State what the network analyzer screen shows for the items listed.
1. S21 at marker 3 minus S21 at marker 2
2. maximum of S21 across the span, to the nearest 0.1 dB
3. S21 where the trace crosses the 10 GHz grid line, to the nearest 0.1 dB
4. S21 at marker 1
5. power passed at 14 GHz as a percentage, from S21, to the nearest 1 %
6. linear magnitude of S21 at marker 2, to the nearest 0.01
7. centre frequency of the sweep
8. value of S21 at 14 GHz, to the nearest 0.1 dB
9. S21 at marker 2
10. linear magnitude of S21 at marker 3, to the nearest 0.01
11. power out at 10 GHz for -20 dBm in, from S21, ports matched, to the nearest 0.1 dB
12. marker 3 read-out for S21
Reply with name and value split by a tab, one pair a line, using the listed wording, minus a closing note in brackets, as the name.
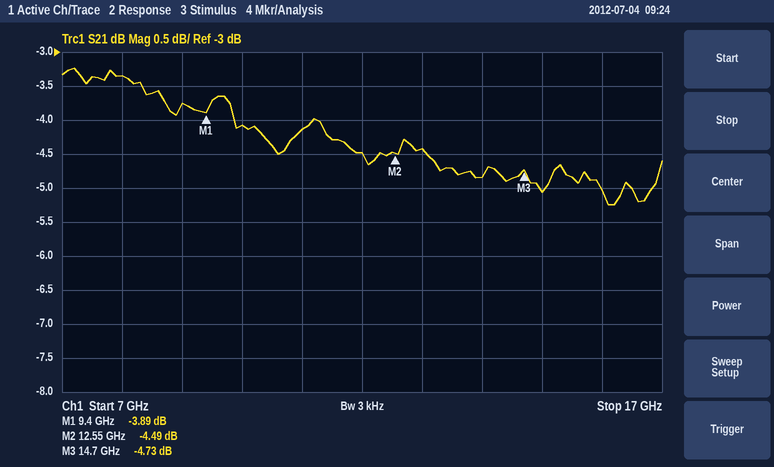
S21 at marker 3 minus S21 at marker 2	-0.24 dB
maximum of S21 across the span, to the nearest 0.1 dB	-3.2 dB
S21 where the trace crosses the 10 GHz grid line, to the nearest 0.1 dB	-4.1 dB
S21 at marker 1	-3.89 dB
power passed at 14 GHz as a percentage, from S21, to the nearest 1 %	33 %
linear magnitude of S21 at marker 2, to the nearest 0.01	0.60
centre frequency of the sweep	12 GHz
value of S21 at 14 GHz, to the nearest 0.1 dB	-4.8 dB
S21 at marker 2	-4.49 dB
linear magnitude of S21 at marker 3, to the nearest 0.01	0.58
power out at 10 GHz for -20 dBm in, from S21, ports matched, to the nearest 0.1 dB	-24.1 dBm
marker 3 read-out for S21	-4.73 dB
